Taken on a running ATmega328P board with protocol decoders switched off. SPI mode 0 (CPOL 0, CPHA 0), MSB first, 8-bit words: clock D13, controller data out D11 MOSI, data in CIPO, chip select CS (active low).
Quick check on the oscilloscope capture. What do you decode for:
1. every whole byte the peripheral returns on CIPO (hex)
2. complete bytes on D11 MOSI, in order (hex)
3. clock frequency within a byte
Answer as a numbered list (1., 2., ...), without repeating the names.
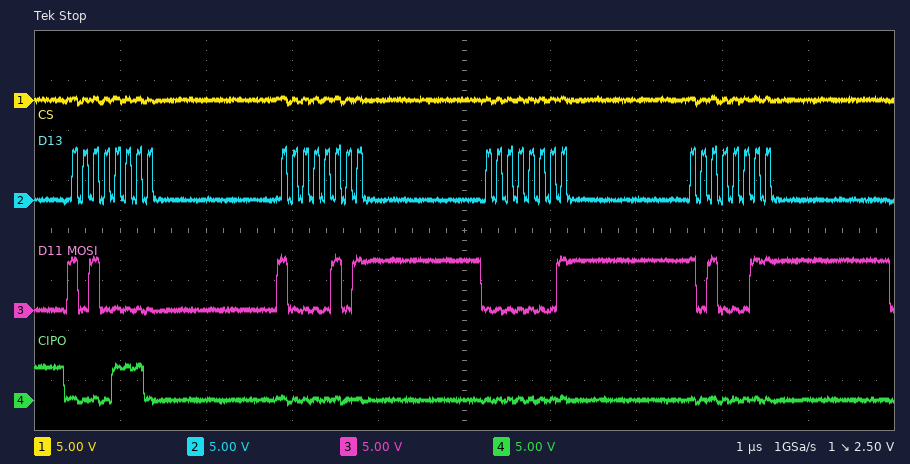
1. 0x0E 0x00 0x00 0x00
2. 0xA0 0x85 0x01 0xA3
3. 8 MHz
